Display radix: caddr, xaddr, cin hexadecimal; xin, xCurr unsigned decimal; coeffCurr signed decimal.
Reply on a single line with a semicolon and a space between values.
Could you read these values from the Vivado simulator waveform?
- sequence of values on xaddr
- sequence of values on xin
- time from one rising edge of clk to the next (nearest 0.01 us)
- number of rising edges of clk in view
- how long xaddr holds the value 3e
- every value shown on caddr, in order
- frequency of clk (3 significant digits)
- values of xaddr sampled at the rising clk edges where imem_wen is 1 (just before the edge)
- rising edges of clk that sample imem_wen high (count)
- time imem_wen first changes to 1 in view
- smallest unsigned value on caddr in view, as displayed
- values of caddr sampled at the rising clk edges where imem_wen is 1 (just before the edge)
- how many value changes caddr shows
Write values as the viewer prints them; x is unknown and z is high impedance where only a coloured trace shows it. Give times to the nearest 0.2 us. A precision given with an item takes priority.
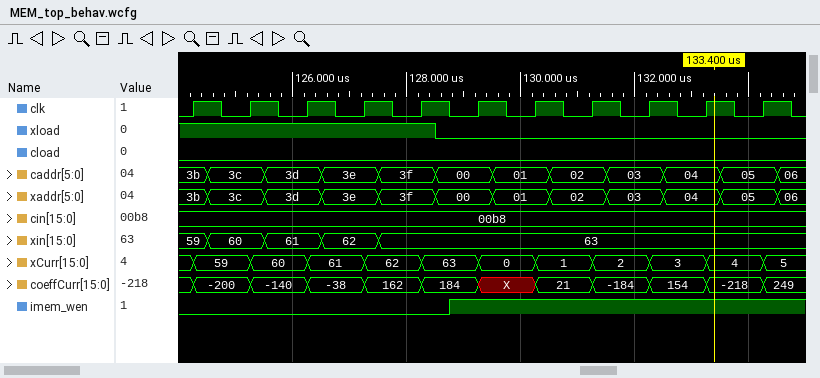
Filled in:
3b, 3c, 3d, 3e, 3f, 00, 01, 02, 03, 04, 05, 06; 59, 60, 61, 62, 63; 1 us; 11; 1 us; 3b, 3c, 3d, 3e, 3f, 00, 01, 02, 03, 04, 05, 06; 1.00 MHz; 00, 01, 02, 03, 04, 05; 6; 128.8 us; 00; 00, 01, 02, 03, 04, 05; 11
